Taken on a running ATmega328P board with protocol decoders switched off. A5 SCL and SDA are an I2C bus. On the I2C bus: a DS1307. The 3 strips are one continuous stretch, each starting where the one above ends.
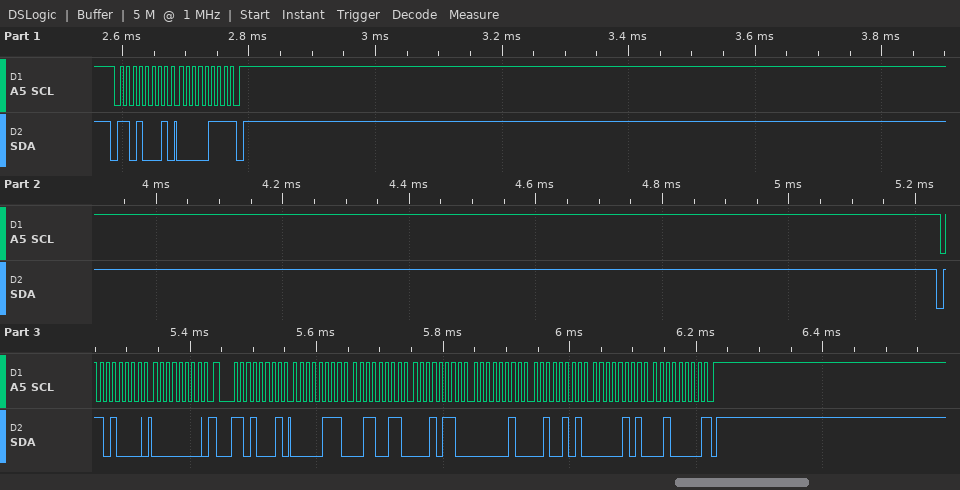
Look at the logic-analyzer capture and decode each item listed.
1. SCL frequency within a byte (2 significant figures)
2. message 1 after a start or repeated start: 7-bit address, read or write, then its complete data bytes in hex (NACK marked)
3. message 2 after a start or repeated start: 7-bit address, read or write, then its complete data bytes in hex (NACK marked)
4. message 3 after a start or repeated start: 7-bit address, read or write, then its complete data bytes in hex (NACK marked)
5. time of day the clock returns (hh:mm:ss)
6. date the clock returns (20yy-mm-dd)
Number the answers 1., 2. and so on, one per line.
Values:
1. 100 kHz
2. 0x68 read: 07 NACK
3. 0x68 write: 00
4. 0x68 read: 07 33 16 02 25 05 20 NACK
5. 16:33:07
6. 2020-05-25
